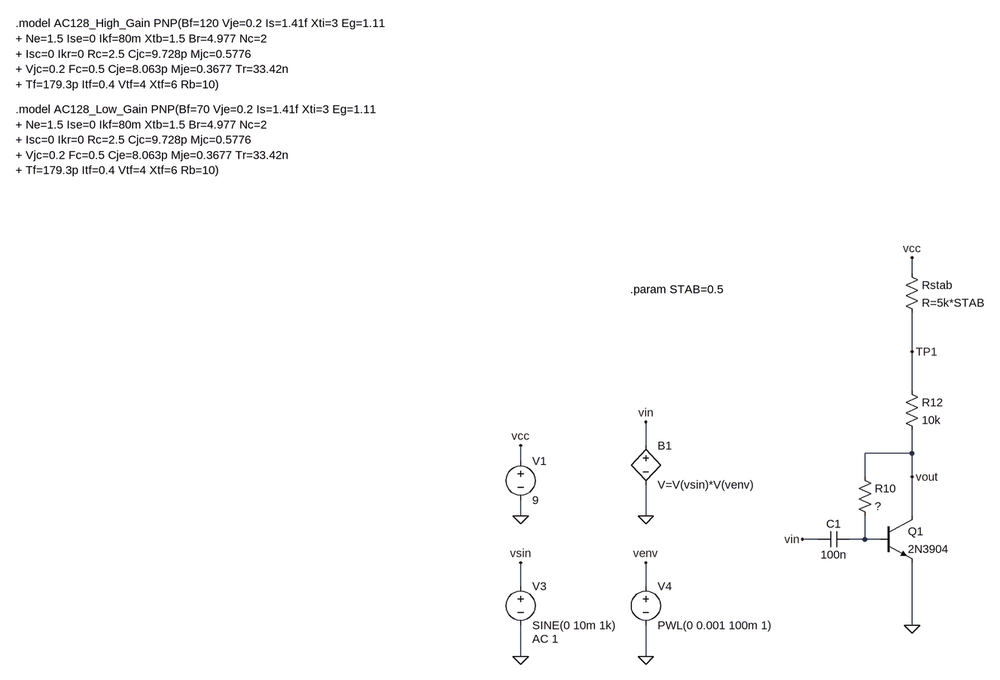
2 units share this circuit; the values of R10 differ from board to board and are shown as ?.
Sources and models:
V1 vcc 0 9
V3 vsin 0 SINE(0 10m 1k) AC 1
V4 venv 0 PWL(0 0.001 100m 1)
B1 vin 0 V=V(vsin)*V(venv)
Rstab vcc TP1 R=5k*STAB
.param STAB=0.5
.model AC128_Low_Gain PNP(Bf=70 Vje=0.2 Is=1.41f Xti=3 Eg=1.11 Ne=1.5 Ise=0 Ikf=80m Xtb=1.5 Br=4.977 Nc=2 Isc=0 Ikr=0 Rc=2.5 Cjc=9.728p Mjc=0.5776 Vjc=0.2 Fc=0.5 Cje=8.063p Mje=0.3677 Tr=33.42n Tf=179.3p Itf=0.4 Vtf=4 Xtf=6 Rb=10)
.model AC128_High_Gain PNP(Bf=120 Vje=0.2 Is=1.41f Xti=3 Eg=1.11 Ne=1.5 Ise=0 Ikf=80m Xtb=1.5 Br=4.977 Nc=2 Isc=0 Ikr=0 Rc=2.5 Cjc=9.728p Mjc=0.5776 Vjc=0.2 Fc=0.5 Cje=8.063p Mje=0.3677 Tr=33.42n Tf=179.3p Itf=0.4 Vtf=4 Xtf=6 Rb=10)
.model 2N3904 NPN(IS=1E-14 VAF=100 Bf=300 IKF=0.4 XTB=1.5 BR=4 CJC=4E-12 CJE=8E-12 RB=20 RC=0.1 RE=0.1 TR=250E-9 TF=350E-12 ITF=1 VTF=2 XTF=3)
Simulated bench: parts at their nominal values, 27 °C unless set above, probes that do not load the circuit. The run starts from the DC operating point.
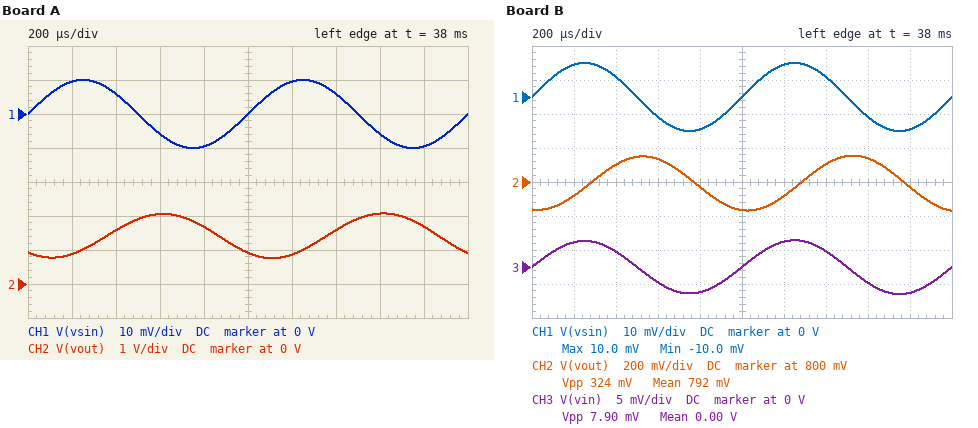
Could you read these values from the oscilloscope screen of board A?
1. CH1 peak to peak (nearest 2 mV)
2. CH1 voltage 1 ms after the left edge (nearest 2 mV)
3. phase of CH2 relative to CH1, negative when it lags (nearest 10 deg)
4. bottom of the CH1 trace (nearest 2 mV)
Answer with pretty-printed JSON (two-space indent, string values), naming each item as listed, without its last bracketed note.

{
  "CH1 peak to peak": "20 mV",
  "CH1 voltage 1 ms after the left edge": "0 V",
  "phase of CH2 relative to CH1, negative when it lags": "-130 deg",
  "bottom of the CH1 trace": "-10 mV"
}
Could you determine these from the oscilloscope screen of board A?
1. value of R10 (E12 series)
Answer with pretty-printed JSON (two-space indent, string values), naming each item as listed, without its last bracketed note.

{
  "value of R10": "390 kΩ"
}
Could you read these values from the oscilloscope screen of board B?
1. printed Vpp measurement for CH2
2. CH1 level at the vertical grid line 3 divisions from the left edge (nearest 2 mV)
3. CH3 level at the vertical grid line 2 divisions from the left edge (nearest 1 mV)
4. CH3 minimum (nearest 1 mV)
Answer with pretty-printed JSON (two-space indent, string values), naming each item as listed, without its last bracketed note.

{
  "printed Vpp measurement for CH2": "324 mV",
  "CH1 level at the vertical grid line 3 divisions from the left edge": "-6 mV",
  "CH3 level at the vertical grid line 2 divisions from the left edge": "2 mV",
  "CH3 minimum": "-4 mV"
}
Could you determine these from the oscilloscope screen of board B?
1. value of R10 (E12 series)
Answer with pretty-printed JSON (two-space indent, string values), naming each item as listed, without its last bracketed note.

{
  "value of R10": "68 kΩ"
}
